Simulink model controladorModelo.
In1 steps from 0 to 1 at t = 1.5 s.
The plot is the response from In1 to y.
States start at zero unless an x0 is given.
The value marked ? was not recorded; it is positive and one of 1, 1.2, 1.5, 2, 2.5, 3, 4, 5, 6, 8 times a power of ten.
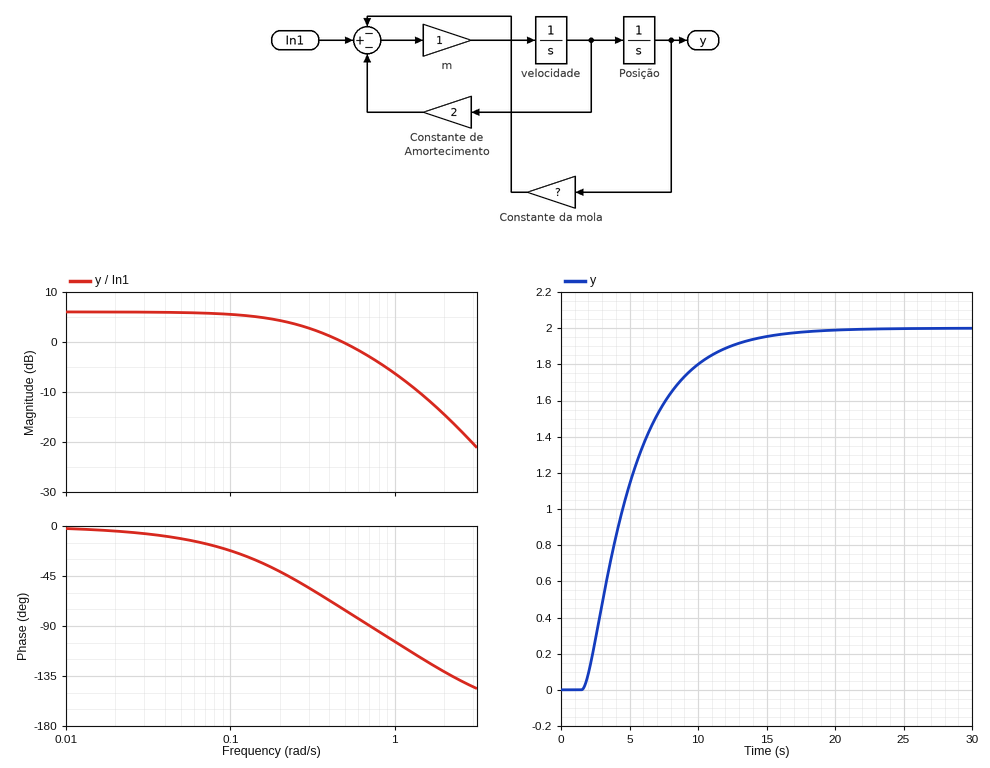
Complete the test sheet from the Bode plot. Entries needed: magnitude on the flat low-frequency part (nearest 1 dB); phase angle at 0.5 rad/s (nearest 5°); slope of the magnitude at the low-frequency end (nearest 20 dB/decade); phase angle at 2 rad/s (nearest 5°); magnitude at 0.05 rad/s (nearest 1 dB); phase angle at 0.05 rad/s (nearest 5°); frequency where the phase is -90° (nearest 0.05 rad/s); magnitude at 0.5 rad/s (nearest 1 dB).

6 dB
-75°
0 dB/decade
-130°
6 dB
-10°
0.70 rad/s
0 dB
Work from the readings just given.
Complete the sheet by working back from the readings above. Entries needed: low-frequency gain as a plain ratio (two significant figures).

2.0
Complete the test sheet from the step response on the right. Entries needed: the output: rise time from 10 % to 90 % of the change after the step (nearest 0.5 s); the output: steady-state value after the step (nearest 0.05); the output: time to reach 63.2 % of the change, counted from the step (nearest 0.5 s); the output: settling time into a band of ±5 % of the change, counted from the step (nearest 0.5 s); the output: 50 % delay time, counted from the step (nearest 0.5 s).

7.5 s
2.00
4.0 s
11.0 s
3.0 s
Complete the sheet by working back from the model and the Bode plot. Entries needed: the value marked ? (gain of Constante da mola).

0.5
